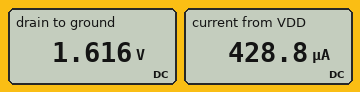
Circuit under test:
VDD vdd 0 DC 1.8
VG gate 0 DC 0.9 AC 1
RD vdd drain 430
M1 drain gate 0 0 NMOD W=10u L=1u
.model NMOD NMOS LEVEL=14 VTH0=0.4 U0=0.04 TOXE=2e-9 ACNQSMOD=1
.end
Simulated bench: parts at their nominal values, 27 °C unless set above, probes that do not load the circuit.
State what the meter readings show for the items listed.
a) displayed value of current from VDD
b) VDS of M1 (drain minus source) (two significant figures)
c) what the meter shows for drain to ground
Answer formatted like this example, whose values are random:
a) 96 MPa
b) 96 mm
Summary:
a) 428.8 µA
b) 1.6 V
c) 1.616 V
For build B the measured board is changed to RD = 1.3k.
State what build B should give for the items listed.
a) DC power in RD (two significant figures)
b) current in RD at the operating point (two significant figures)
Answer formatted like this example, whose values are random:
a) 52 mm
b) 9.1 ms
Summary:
a) 230 µW
b) 420 µA
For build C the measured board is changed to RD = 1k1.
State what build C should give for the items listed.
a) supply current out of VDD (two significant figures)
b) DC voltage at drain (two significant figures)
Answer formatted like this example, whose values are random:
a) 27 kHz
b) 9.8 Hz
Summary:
a) 420 µA
b) 1.3 V
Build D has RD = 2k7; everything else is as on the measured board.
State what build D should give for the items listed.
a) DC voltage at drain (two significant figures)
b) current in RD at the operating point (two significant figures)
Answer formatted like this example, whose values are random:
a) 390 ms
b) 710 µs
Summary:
a) 720 mV
b) 400 µA
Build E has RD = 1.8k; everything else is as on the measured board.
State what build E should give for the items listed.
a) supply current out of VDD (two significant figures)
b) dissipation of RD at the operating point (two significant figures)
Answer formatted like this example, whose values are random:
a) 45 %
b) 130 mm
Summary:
a) 410 µA
b) 310 µW
